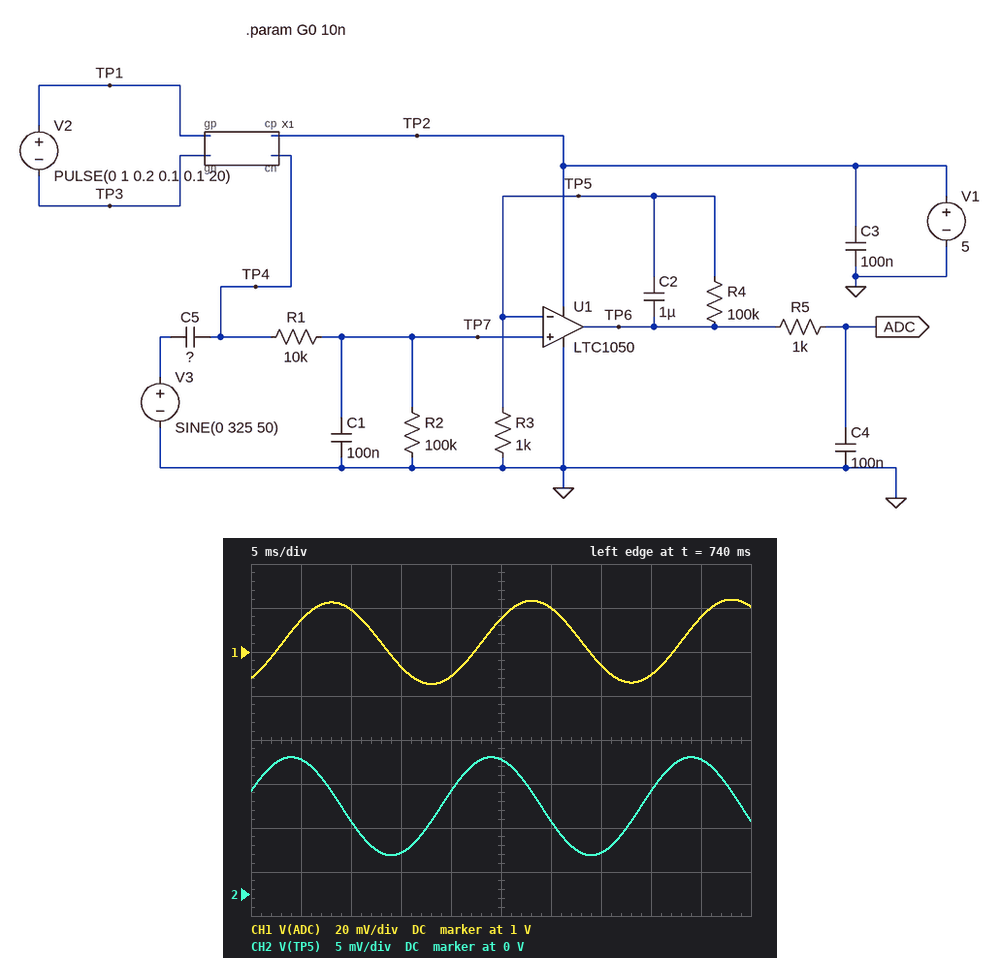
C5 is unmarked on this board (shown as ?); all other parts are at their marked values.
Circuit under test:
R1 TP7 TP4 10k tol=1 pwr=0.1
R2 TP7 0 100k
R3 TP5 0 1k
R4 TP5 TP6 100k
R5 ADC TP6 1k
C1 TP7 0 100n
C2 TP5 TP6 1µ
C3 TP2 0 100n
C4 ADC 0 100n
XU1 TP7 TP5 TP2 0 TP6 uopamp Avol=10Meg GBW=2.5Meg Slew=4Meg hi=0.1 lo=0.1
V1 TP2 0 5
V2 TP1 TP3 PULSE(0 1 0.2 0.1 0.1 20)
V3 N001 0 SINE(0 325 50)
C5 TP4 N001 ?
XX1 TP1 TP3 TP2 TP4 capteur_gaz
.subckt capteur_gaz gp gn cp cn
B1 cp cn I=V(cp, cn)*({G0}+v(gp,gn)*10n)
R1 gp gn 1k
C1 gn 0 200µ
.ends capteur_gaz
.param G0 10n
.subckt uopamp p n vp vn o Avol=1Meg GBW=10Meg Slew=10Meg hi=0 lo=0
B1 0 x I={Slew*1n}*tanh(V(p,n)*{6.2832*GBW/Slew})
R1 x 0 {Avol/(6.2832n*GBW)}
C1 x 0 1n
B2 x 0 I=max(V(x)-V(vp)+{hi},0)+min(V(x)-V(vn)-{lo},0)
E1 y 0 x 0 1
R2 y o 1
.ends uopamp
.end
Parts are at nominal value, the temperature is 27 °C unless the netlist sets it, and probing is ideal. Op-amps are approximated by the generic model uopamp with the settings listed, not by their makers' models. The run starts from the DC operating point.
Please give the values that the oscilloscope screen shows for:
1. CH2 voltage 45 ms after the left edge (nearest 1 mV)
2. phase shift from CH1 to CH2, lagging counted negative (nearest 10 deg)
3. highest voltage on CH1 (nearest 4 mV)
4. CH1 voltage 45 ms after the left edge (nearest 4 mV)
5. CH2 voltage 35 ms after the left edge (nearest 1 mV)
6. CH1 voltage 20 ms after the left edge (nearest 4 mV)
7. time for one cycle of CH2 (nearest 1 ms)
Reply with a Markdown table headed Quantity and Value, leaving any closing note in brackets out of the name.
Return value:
| Quantity | Value |
|---|---|
| CH2 voltage 45 ms after the left edge | 15 mV |
| phase shift from CH1 to CH2, lagging counted negative | 70 deg |
| highest voltage on CH1 | 1.024 V |
| CH1 voltage 45 ms after the left edge | 1.016 V |
| CH2 voltage 35 ms after the left edge | 5 mV |
| CH1 voltage 20 ms after the left edge | 988 mV |
| time for one cycle of CH2 | 20 ms |
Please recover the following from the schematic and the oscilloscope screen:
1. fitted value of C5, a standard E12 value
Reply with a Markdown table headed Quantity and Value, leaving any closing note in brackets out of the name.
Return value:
| Quantity | Value |
|---|---|
| fitted value of C5, a standard E12 value | 1.8 pF |
